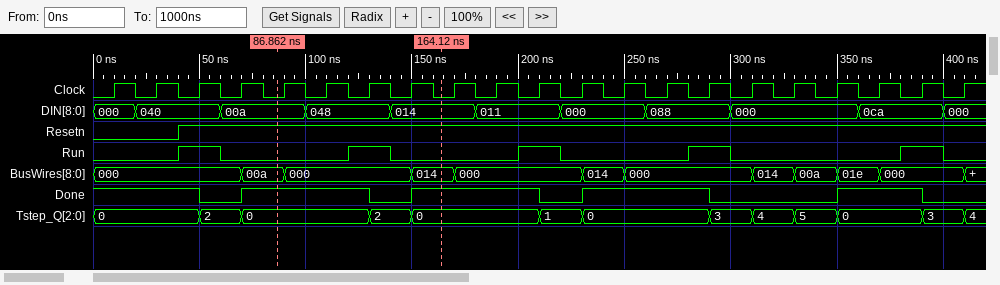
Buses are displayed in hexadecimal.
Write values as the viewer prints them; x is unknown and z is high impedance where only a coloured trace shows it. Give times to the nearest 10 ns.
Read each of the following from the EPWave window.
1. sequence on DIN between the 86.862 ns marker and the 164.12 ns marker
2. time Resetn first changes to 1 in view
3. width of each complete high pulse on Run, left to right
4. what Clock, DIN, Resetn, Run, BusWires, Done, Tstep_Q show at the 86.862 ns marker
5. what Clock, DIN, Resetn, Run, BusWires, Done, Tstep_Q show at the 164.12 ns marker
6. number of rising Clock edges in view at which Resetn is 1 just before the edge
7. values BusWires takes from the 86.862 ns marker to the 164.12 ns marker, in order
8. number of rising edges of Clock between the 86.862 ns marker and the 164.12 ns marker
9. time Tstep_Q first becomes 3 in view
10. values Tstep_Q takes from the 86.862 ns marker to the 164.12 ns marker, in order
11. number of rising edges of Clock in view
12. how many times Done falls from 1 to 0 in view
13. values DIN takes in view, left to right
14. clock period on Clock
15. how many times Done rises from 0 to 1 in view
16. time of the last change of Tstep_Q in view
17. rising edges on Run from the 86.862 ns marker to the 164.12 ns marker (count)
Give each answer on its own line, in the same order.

00a, 048, 014
40 ns
20 ns, 20 ns, 20 ns, 20 ns, 20 ns
Clock=0, DIN=00a, Resetn=1, Run=0, BusWires=00a, Done=1, Tstep_Q=0
Clock=0, DIN=014, Resetn=1, Run=0, BusWires=014, Done=1, Tstep_Q=0
19
00a, 000, 014
4
290 ns
0, 2, 0
21
5
000, 040, 00a, 048, 014, 011, 000, 088, 000, 0ca, 000
20 ns
4
410 ns
1
